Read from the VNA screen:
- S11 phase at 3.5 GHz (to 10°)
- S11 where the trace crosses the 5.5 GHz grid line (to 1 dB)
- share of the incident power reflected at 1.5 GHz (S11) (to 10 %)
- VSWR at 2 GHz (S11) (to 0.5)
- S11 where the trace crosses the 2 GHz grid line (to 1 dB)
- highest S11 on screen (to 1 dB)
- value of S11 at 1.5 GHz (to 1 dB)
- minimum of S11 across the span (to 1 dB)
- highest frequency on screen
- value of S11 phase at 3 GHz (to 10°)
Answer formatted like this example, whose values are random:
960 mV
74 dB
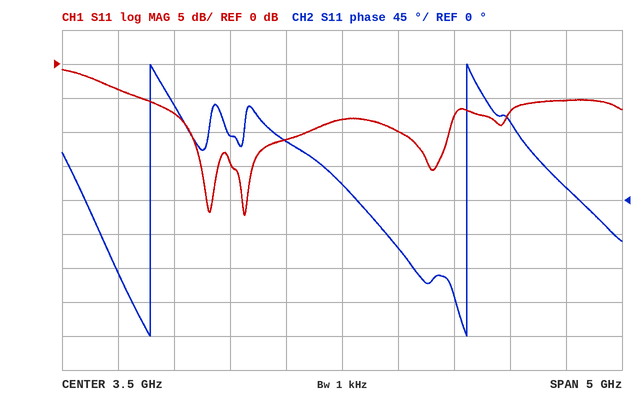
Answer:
20°
-5 dB
40 %
2.5
-7 dB
-1 dB
-4 dB
-22 dB
6 GHz
80°
